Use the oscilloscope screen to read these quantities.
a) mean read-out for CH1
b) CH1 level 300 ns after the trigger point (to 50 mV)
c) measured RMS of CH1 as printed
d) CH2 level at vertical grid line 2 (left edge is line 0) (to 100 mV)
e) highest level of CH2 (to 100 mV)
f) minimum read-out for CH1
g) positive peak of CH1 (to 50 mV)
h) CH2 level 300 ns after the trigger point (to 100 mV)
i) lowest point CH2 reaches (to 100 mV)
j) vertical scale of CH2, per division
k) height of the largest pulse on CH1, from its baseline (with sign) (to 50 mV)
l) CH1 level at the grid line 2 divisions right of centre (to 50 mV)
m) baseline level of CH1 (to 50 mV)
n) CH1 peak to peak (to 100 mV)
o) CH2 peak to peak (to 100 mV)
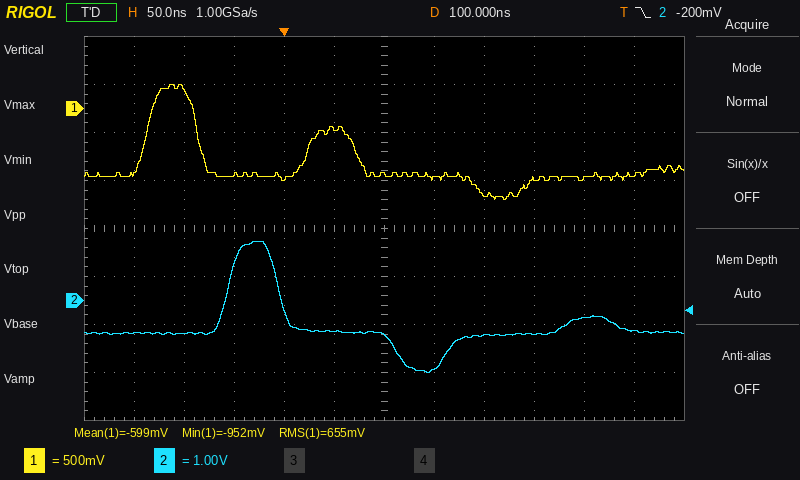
-599 mV
-750 mV
655 mV
-700 mV
1.2 V
-952 mV
250 mV
-400 mV
-1.5 V
1 V
+950 mV
-900 mV
-700 mV
1.20 V
2.7 V
